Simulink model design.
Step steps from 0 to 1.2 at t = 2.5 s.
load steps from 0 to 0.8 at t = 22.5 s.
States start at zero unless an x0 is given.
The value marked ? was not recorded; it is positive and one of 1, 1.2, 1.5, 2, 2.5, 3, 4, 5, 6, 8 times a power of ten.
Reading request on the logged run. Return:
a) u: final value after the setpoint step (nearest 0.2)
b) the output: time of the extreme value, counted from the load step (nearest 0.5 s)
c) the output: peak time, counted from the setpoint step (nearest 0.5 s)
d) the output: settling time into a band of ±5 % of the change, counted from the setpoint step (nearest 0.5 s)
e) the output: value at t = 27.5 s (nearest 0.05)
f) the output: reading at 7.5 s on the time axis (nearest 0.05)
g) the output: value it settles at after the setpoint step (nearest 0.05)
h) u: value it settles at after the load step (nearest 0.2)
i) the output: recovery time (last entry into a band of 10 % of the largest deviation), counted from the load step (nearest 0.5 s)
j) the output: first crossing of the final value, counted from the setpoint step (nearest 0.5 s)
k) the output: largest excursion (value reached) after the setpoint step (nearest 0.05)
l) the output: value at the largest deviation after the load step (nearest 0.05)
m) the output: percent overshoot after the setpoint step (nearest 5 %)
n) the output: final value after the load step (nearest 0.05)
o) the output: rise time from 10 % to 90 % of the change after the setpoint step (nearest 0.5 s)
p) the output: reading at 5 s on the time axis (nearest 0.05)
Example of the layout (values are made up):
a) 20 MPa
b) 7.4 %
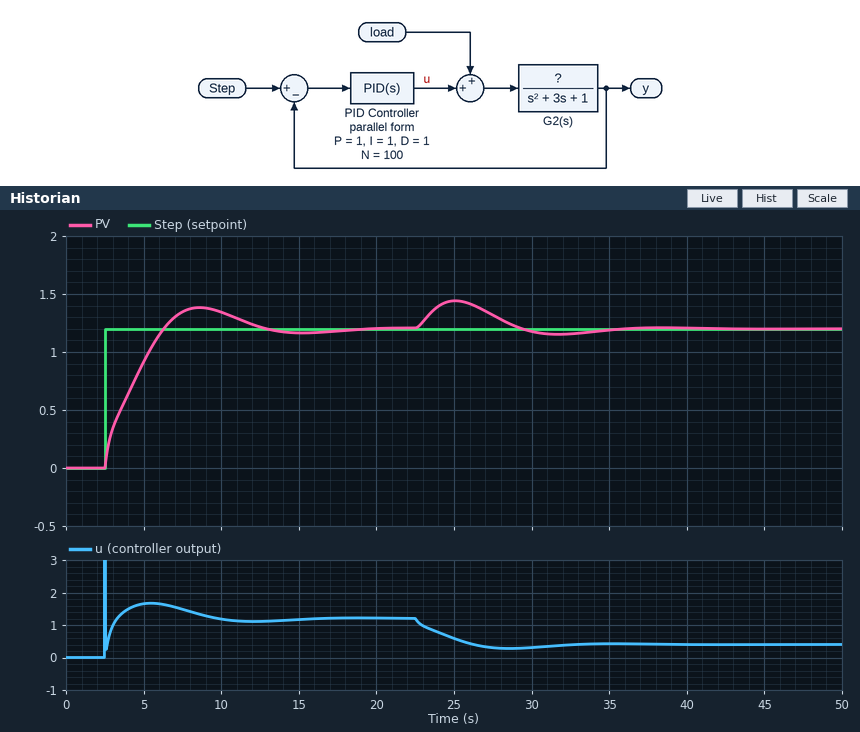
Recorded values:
a) 1.2
b) 2.5 s
c) 6.0 s
d) 9.0 s
e) 1.30
f) 1.35
g) 1.20
h) 0.4
i) 11.5 s
j) 4.0 s
k) 1.40
l) 1.45
m) 15 %
n) 1.20
o) 3.0 s
p) 0.90
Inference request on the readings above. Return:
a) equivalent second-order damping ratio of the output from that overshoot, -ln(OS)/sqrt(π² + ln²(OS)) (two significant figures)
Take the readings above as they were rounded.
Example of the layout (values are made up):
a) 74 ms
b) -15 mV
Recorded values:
a) 0.52
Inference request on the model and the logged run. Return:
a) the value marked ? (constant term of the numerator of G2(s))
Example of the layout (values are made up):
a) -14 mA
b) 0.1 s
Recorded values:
a) 1
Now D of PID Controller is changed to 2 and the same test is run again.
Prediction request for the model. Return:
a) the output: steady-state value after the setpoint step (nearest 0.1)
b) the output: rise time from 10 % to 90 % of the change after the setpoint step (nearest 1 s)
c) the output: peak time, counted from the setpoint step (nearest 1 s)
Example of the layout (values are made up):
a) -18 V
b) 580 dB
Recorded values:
a) 1.2
b) 4 s
c) 7 s
